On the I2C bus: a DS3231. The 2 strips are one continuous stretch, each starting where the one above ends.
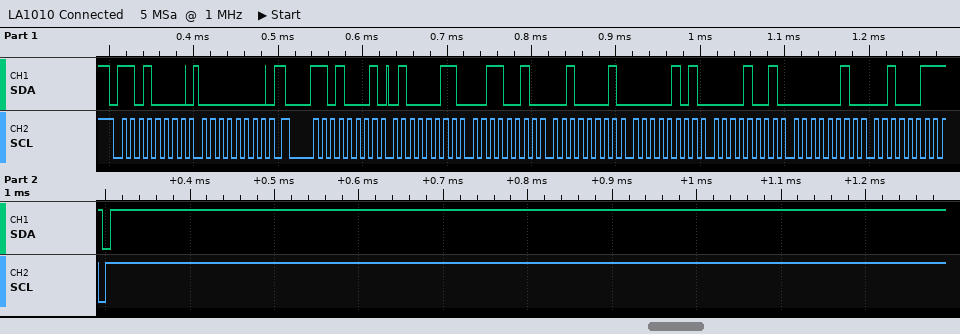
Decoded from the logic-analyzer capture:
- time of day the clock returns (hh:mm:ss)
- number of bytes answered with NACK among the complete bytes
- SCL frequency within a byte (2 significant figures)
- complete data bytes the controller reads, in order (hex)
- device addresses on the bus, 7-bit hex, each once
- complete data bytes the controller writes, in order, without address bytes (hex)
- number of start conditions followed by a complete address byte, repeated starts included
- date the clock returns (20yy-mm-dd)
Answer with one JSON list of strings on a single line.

["21:32:43", "1", "100 kHz", "43 32 21 05 09 02 23", "0x68", "00", "2", "2023-02-09"]
